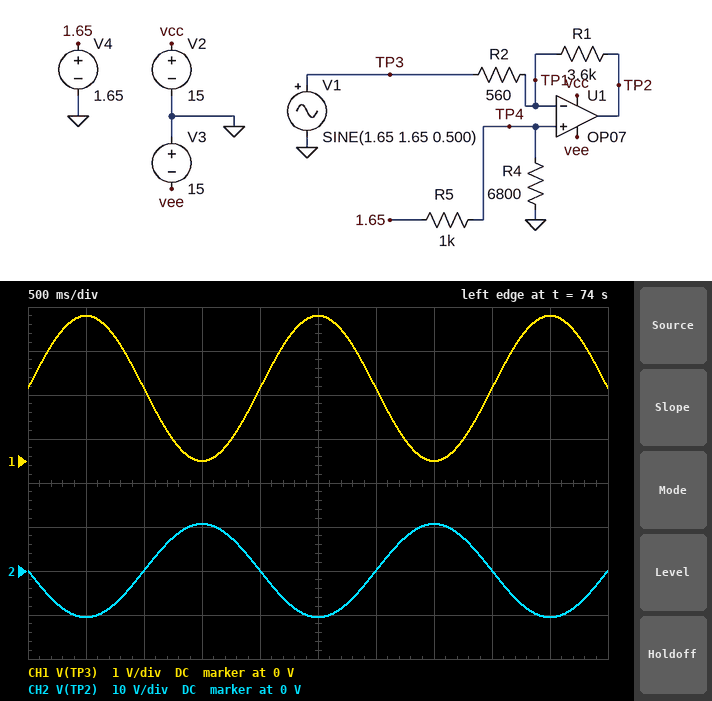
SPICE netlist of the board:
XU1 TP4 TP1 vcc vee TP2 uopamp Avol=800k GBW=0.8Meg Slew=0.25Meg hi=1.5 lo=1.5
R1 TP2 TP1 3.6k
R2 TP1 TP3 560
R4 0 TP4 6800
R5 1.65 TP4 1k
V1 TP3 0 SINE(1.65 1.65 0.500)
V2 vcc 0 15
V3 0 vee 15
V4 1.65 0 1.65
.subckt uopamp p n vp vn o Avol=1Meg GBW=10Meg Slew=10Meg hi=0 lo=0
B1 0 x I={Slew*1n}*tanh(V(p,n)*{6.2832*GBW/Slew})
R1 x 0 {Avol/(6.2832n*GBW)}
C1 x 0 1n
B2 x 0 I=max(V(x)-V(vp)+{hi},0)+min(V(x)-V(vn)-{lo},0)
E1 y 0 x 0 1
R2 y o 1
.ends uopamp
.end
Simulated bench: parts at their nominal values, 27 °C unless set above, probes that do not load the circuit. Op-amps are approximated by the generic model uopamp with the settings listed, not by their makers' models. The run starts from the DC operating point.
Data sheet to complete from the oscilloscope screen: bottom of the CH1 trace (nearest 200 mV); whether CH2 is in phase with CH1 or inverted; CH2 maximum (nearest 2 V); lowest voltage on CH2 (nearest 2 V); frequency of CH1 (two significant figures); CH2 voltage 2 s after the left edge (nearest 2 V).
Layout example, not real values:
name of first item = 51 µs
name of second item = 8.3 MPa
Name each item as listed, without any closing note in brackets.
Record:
bottom of the CH1 trace = 0 V
whether CH2 is in phase with CH1 or inverted = inverted
CH2 maximum = 10 V
lowest voltage on CH2 = -10 V
frequency of CH1 = 500 mHz
CH2 voltage 2 s after the left edge = 0 V
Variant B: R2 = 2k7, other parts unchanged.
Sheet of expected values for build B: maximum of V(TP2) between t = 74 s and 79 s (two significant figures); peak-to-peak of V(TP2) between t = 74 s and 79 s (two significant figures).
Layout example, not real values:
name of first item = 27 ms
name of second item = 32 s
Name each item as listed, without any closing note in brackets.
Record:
maximum of V(TP2) between t = 74 s and 79 s = 3.4 V
peak-to-peak of V(TP2) between t = 74 s and 79 s = 4.4 V
